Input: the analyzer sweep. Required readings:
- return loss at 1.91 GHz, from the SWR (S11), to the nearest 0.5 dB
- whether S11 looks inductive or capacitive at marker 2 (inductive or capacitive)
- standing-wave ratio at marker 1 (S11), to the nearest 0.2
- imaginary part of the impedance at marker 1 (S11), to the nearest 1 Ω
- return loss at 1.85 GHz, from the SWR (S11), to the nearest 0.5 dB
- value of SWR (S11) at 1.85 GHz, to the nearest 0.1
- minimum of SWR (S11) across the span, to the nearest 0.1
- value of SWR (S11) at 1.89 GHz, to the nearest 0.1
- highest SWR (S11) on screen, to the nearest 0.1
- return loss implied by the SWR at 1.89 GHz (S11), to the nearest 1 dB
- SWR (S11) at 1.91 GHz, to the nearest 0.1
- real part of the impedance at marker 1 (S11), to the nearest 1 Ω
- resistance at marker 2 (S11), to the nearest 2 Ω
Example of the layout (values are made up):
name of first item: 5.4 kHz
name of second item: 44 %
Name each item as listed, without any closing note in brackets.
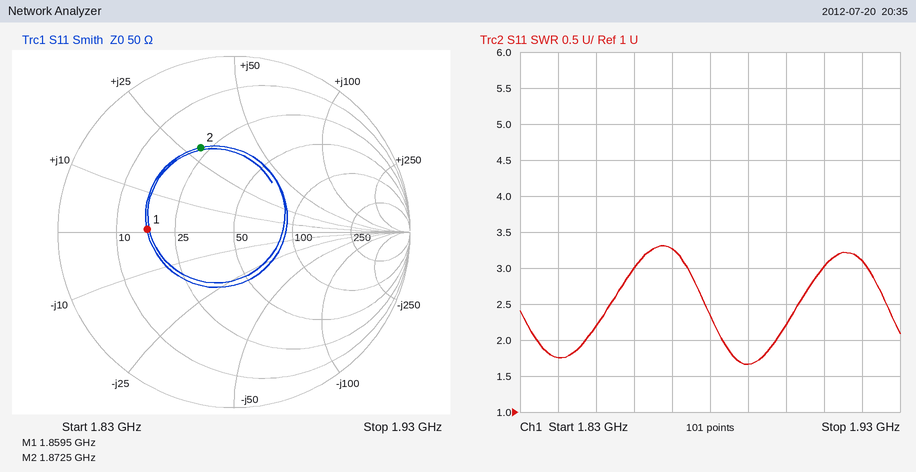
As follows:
return loss at 1.91 GHz, from the SWR (S11), to the nearest 0.5 dB: 6.0 dB
whether S11 looks inductive or capacitive at marker 2: inductive
standing-wave ratio at marker 1 (S11), to the nearest 0.2: 3.0
imaginary part of the impedance at marker 1 (S11), to the nearest 1 Ω: +1 Ω
return loss at 1.85 GHz, from the SWR (S11), to the nearest 0.5 dB: 8.5 dB
value of SWR (S11) at 1.85 GHz, to the nearest 0.1: 2.2
minimum of SWR (S11) across the span, to the nearest 0.1: 1.7
value of SWR (S11) at 1.89 GHz, to the nearest 0.1: 1.7
highest SWR (S11) on screen, to the nearest 0.1: 3.3
return loss implied by the SWR at 1.89 GHz (S11), to the nearest 1 dB: 12 dB
SWR (S11) at 1.91 GHz, to the nearest 0.1: 3.0
real part of the impedance at marker 1 (S11), to the nearest 1 Ω: 17 Ω
resistance at marker 2 (S11), to the nearest 2 Ω: 22 Ω
